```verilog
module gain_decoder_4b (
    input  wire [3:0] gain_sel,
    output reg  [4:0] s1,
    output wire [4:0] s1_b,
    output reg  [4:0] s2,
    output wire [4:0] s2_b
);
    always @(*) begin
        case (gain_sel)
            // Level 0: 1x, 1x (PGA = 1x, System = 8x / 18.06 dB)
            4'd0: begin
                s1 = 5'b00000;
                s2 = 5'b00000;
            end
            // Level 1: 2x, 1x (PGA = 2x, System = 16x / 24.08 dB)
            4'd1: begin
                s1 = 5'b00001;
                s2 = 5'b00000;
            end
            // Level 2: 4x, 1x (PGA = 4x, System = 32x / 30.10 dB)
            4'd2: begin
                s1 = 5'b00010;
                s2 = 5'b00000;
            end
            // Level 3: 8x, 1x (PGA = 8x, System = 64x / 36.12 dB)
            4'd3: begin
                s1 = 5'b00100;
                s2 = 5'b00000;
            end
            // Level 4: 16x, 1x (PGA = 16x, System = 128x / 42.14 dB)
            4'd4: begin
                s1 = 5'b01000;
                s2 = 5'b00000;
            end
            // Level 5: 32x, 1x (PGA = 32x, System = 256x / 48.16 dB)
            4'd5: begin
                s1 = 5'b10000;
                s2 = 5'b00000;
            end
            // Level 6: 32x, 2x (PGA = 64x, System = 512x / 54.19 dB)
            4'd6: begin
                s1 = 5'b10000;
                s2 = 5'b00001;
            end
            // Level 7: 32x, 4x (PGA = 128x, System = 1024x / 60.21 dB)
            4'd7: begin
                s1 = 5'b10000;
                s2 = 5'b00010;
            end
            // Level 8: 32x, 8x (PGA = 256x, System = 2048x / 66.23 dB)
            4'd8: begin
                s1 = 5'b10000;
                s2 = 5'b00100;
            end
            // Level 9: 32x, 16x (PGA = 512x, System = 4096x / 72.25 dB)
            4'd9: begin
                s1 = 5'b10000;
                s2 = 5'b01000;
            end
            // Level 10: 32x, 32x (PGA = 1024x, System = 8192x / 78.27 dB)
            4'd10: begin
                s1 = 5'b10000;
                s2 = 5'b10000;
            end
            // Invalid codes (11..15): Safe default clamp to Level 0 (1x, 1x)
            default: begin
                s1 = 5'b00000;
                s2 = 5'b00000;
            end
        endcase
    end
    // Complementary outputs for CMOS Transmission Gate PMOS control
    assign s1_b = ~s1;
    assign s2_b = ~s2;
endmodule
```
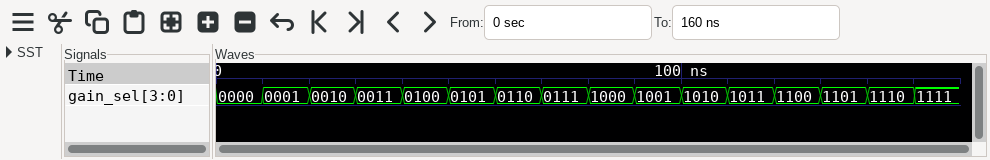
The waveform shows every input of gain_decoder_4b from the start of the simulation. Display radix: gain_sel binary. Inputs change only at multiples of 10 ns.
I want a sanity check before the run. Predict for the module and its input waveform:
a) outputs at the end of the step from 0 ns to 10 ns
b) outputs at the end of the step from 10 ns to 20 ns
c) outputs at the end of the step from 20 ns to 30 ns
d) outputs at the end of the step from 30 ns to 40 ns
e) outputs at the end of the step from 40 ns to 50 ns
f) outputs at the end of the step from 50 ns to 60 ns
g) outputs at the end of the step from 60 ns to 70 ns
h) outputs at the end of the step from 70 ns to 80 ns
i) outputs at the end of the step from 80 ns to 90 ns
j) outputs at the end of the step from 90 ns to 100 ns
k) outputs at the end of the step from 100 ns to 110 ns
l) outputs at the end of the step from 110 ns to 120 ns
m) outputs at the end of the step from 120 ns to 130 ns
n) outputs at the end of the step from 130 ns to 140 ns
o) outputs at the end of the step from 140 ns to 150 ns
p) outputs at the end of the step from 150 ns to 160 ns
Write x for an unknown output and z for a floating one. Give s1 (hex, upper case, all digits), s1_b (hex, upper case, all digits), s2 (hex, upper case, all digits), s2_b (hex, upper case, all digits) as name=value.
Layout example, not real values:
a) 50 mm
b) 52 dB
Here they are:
a) s1=00, s1_b=1F, s2=00, s2_b=1F
b) s1=01, s1_b=1E, s2=00, s2_b=1F
c) s1=02, s1_b=1D, s2=00, s2_b=1F
d) s1=04, s1_b=1B, s2=00, s2_b=1F
e) s1=08, s1_b=17, s2=00, s2_b=1F
f) s1=10, s1_b=0F, s2=00, s2_b=1F
g) s1=10, s1_b=0F, s2=01, s2_b=1E
h) s1=10, s1_b=0F, s2=02, s2_b=1D
i) s1=10, s1_b=0F, s2=04, s2_b=1B
j) s1=10, s1_b=0F, s2=08, s2_b=17
k) s1=10, s1_b=0F, s2=10, s2_b=0F
l) s1=00, s1_b=1F, s2=00, s2_b=1F
m) s1=00, s1_b=1F, s2=00, s2_b=1F
n) s1=00, s1_b=1F, s2=00, s2_b=1F
o) s1=00, s1_b=1F, s2=00, s2_b=1F
p) s1=00, s1_b=1F, s2=00, s2_b=1F
